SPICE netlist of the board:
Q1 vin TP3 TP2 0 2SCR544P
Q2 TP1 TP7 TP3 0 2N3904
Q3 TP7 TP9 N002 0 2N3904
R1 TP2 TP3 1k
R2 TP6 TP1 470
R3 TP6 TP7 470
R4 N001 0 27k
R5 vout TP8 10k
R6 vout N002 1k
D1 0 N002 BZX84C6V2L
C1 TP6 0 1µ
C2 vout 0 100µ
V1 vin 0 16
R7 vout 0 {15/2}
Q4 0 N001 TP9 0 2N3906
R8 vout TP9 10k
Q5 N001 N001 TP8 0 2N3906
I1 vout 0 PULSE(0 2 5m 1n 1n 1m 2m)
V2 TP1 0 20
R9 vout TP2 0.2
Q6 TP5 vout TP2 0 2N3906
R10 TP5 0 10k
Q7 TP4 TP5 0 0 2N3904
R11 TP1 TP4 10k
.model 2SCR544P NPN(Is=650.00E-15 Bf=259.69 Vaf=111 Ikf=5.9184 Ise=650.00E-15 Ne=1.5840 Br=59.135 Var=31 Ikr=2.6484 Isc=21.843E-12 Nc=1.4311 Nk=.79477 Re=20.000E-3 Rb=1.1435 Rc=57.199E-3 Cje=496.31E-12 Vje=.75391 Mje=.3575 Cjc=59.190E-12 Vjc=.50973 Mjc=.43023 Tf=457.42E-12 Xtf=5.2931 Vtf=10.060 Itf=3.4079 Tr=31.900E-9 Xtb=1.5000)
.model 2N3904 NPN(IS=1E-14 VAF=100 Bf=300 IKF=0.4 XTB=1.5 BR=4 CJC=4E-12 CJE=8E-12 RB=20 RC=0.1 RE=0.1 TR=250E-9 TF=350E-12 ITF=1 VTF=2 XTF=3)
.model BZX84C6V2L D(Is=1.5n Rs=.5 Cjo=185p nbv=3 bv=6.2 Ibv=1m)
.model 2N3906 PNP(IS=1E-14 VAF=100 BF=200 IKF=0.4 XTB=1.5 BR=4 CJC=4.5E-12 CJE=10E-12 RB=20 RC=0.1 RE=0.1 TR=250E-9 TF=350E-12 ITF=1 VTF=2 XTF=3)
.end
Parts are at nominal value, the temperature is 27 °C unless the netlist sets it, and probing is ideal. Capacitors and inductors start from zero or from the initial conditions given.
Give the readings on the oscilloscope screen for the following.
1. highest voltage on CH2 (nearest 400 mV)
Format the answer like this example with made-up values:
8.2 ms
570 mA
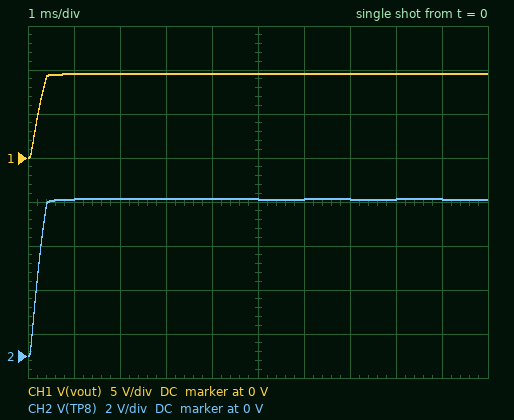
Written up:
7.2 V
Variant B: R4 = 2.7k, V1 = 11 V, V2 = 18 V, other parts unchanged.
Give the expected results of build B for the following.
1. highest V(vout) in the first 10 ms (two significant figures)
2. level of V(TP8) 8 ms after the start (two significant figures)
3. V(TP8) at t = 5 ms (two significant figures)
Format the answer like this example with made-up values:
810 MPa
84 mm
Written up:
11 V
2.7 V
2.8 V
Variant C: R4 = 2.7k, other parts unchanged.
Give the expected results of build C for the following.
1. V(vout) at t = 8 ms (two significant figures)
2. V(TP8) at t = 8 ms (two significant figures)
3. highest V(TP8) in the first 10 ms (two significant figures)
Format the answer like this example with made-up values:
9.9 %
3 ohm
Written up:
15 V
3.7 V
3.8 V
